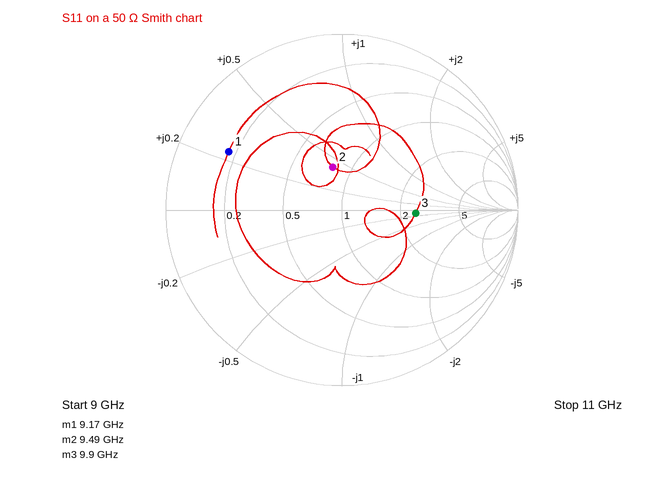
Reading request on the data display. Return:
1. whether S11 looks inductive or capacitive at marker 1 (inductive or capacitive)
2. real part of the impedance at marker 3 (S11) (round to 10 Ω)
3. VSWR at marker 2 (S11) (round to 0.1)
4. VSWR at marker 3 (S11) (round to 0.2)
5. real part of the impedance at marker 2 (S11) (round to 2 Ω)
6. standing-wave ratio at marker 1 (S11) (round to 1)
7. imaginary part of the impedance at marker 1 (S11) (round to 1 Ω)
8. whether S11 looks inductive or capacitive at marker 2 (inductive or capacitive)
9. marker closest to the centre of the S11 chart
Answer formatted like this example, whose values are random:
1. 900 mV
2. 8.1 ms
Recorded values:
1. inductive
2. 120 Ω
3. 1.7
4. 2.4
5. 40 Ω
6. 6
7. +12 Ω
8. inductive
9. marker 2
